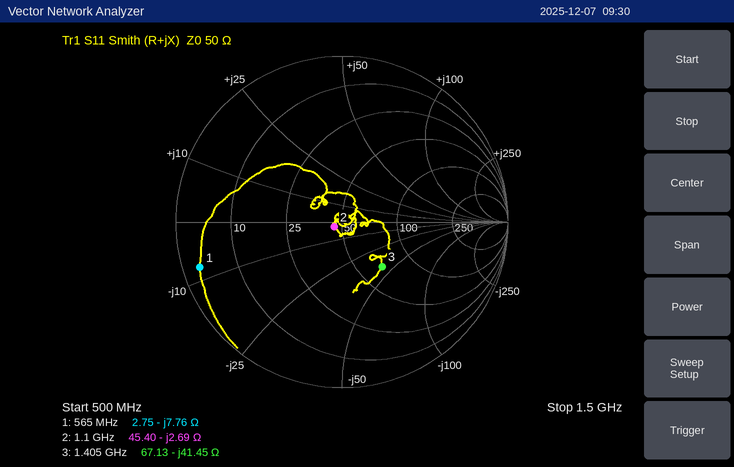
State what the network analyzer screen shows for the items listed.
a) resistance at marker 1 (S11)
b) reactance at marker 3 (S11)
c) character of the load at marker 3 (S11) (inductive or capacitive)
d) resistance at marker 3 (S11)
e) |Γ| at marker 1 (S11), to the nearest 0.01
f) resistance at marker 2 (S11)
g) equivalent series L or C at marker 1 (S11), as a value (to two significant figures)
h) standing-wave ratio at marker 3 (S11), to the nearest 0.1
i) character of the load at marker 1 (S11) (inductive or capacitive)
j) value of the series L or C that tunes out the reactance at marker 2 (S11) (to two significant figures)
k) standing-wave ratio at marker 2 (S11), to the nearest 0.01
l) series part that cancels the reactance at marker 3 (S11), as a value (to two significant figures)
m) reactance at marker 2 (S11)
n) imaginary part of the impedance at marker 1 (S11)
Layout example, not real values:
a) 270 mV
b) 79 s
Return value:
a) 2.75 Ω
b) -41.45 Ω
c) capacitive
d) 67.13 Ω
e) 0.90
f) 45.40 Ω
g) 36 pF
h) 2.1
i) capacitive
j) 390 pH
k) 1.12
l) 4.7 nH
m) -2.69 Ω
n) -7.76 Ω
